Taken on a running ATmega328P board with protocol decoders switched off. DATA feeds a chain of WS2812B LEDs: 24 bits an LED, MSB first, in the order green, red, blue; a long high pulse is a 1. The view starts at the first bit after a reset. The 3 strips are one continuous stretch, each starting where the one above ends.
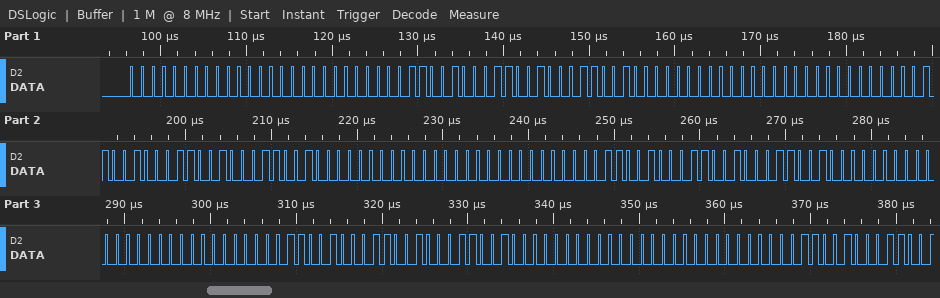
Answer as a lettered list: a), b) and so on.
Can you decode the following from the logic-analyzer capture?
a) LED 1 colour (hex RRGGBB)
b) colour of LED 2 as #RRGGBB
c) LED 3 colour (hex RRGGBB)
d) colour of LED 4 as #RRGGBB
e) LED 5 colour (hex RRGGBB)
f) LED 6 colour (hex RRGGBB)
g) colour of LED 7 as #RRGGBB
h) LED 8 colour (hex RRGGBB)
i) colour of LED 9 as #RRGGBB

a) #000000
b) #323232
c) #000000
d) #323232
e) #000000
f) #323232
g) #000000
h) #323232
i) #000000
